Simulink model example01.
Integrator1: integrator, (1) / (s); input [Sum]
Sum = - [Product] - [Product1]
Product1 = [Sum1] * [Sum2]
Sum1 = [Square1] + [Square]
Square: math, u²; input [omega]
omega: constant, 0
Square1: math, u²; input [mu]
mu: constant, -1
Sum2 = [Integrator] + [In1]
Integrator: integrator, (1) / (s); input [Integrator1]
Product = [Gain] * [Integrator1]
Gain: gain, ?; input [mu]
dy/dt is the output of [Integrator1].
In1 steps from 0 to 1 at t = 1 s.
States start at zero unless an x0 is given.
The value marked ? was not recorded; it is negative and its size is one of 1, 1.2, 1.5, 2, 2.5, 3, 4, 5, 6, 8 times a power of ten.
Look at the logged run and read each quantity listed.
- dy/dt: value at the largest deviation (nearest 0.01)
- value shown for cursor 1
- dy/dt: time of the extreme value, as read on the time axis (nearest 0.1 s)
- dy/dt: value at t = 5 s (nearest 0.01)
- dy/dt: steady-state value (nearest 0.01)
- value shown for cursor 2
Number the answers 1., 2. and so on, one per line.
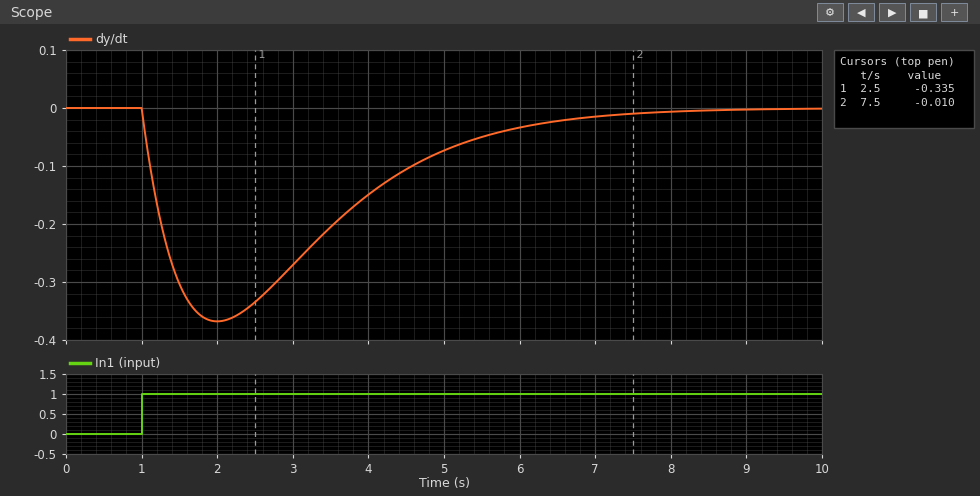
1. -0.37
2. -0.335
3. 2.0 s
4. -0.07
5. 0.00
6. -0.010
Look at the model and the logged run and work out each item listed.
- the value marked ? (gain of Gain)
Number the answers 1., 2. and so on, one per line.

1. -2
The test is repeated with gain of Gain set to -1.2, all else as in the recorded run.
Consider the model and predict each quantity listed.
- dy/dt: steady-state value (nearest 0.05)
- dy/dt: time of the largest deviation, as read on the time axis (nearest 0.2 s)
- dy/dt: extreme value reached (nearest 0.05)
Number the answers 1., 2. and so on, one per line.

1. 0.00
2. 2.2 s
3. -0.50
